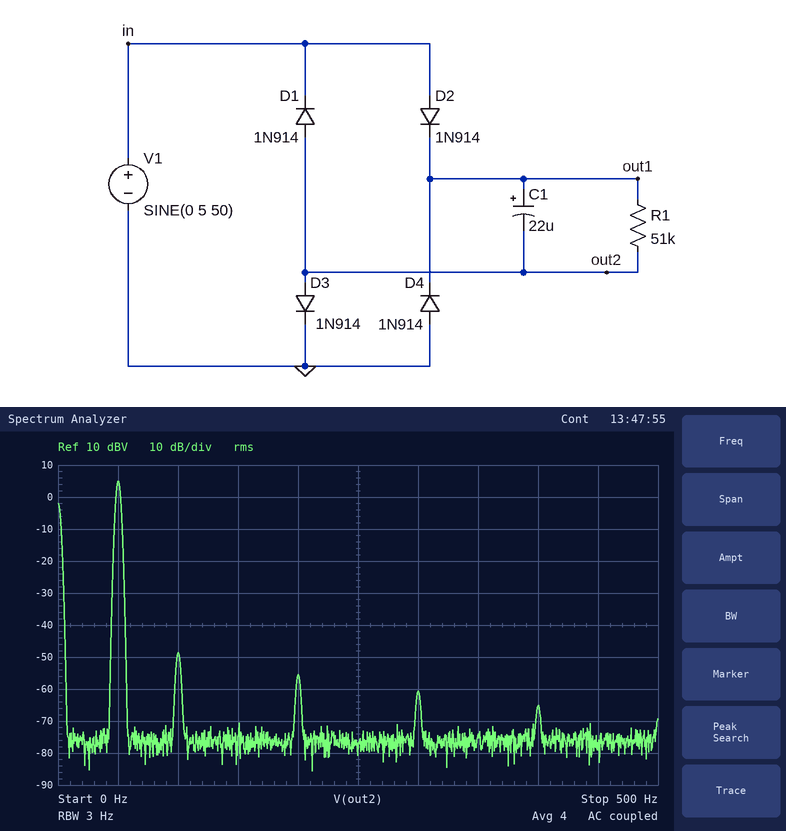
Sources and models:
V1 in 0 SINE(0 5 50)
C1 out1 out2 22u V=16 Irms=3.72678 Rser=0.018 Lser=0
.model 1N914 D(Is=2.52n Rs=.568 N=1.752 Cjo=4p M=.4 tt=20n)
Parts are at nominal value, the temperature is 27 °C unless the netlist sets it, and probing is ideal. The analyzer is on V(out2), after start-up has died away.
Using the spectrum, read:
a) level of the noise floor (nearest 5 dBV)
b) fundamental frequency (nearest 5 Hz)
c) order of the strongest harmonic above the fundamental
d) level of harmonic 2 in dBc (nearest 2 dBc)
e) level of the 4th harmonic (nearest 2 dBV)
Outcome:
-75 dBV
50 Hz
2
-54 dBc
-56 dBV
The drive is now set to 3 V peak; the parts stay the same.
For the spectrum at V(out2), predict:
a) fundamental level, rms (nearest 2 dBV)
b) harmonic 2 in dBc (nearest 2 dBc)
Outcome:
0 dBV
-56 dBc
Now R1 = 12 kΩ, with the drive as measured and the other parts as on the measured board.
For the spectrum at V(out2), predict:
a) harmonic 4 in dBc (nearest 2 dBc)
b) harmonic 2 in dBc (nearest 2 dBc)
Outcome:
-48 dBc
-42 dBc
